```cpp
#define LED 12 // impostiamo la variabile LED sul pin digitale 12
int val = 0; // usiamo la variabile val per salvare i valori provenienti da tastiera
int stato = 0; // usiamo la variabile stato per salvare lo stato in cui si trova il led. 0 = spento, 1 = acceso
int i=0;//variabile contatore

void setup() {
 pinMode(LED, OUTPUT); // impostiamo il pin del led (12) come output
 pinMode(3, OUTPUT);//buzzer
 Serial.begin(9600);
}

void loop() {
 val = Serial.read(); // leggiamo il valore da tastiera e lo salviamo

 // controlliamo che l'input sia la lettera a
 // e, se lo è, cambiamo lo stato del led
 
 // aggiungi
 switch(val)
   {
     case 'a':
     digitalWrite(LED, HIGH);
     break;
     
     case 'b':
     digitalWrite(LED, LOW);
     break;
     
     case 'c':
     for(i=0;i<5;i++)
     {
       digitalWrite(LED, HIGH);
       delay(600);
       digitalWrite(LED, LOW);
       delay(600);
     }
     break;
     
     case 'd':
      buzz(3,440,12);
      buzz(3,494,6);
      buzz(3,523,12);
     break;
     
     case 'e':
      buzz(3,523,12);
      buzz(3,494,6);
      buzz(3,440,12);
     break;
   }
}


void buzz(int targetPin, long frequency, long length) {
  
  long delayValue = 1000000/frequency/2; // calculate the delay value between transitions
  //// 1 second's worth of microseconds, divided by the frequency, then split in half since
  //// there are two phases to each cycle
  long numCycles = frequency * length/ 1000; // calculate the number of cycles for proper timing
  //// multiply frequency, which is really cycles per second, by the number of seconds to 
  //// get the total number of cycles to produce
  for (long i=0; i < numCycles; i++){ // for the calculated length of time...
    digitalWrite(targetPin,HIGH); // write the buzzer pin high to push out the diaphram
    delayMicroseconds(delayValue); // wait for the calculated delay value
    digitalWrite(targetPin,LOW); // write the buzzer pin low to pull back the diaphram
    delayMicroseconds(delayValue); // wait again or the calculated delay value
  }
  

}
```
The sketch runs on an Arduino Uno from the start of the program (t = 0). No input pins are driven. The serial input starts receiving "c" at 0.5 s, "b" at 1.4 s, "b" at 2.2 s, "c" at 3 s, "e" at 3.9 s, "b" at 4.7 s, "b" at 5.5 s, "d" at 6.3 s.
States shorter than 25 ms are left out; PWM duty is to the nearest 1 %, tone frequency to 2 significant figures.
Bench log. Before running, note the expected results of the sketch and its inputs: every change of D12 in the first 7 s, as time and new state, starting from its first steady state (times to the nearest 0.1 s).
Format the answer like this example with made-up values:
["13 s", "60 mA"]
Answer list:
["0 s low; 0.5 s high; 1.1 s low; 1.7 s high; 2.3 s low; 2.9 s high; 3.5 s low; 4.1 s high; 4.7 s low; 5.3 s high; 5.9 s low; 6.5 s high"]
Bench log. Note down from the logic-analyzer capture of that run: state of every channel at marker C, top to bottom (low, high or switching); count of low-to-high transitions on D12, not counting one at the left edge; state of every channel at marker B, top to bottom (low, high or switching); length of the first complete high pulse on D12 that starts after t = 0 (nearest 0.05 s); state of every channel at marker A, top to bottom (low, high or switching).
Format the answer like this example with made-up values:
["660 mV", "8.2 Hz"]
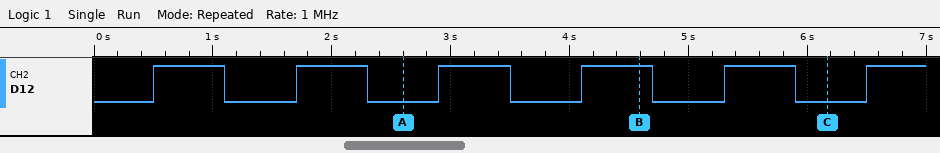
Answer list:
["D12 low", "6", "D12 high", "0.60 s", "D12 low"]
